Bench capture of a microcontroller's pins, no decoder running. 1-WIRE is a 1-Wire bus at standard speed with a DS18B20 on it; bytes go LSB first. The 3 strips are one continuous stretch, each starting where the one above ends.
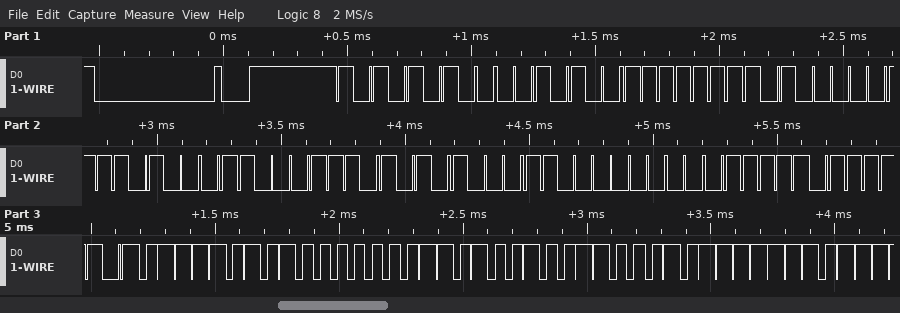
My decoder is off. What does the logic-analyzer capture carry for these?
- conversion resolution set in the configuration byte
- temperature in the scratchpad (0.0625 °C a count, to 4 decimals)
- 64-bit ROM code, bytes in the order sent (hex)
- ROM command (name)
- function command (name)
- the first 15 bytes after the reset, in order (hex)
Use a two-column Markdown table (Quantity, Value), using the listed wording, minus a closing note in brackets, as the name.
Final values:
| Quantity | Value |
|---|---|
| conversion resolution set in the configuration byte | 12 bits |
| temperature in the scratchpad | 21.8750 °C |
| 64-bit ROM code, bytes in the order sent | 28 FF 82 8B 71 15 03 F8 |
| ROM command | Match ROM |
| function command | Read Scratchpad |
| the first 15 bytes after the reset, in order | 55 28 FF 82 8B 71 15 03 F8 BE 5E 01 4B 46 7F |
